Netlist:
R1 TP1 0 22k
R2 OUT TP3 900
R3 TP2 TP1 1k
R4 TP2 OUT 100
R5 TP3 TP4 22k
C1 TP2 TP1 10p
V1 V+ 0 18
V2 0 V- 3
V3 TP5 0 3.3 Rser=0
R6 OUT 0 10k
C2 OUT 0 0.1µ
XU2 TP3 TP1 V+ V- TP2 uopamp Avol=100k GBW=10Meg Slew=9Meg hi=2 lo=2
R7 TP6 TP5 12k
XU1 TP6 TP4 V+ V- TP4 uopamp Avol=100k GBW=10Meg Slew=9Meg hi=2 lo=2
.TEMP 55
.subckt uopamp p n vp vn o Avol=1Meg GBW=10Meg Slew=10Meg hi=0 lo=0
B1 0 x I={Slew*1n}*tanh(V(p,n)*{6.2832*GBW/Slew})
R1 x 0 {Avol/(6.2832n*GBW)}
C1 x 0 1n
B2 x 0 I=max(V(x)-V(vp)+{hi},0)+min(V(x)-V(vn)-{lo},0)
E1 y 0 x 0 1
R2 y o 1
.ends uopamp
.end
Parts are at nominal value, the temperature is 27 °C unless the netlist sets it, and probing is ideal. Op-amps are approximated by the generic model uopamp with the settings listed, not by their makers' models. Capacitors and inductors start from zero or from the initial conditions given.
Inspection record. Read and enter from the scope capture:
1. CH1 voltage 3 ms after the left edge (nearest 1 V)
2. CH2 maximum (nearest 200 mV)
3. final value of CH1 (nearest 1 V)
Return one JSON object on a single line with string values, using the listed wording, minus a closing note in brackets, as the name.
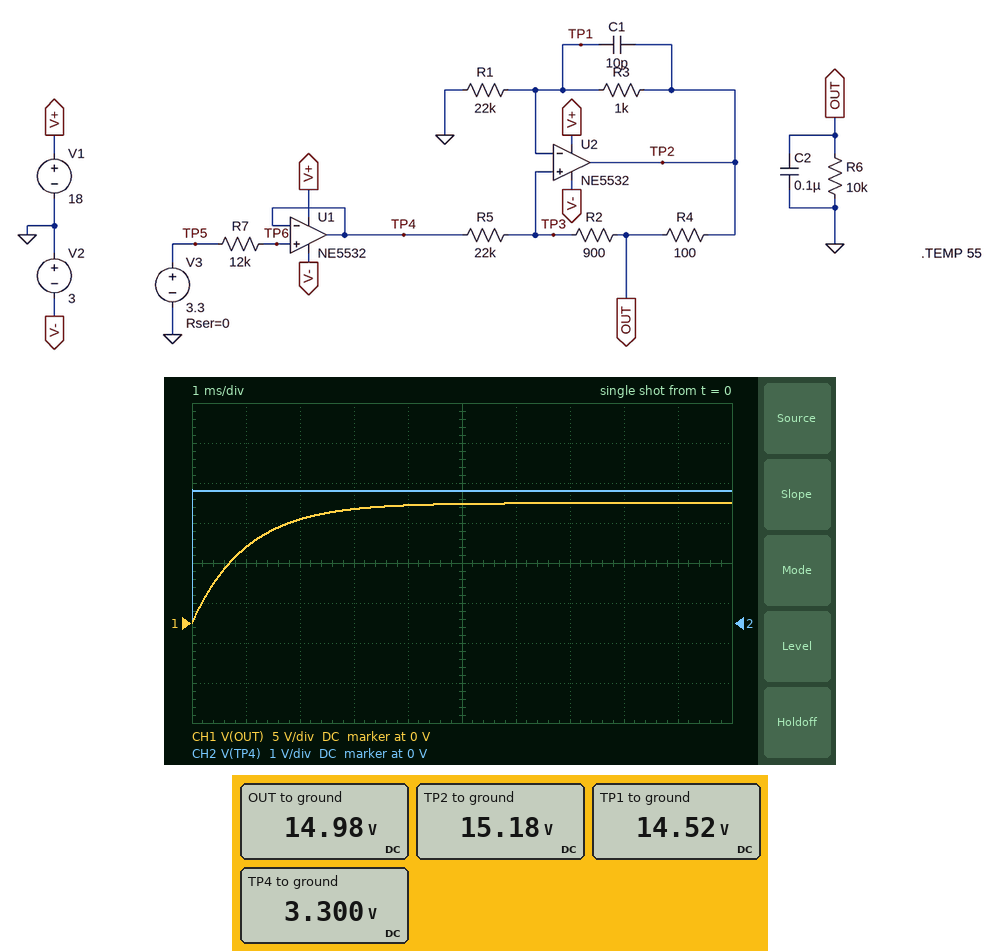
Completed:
{"CH1 voltage 3 ms after the left edge": "14 V", "CH2 maximum": "3.4 V", "final value of CH1": "15 V"}
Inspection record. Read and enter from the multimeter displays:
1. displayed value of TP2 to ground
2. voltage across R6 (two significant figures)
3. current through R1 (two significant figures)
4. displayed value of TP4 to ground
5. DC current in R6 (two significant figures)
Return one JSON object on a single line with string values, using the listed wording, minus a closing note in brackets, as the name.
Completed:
{"displayed value of TP2 to ground": "15.18 V", "voltage across R6": "15 V", "current through R1": "660 µA", "displayed value of TP4 to ground": "3.300 V", "DC current in R6": "1.5 mA"}
